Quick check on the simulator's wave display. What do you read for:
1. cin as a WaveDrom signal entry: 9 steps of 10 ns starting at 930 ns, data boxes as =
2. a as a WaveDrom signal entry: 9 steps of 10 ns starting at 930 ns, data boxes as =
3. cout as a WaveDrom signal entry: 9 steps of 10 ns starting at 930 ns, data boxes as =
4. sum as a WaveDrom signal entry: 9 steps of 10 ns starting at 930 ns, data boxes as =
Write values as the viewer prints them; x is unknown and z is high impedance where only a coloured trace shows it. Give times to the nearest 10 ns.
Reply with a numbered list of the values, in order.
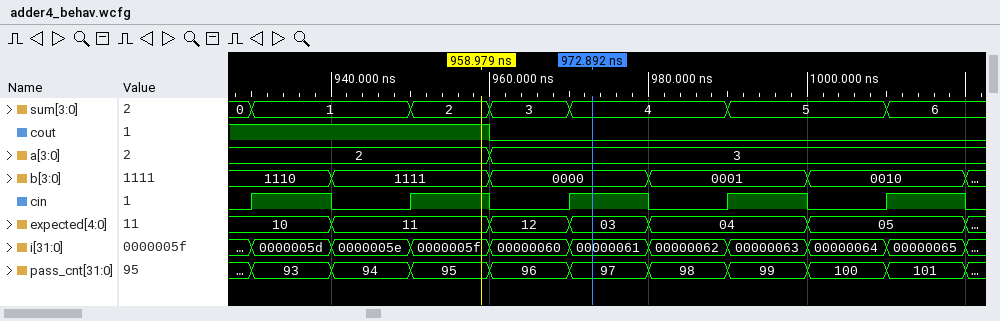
1. {name: 'cin', wave: '101010101'}
2. {name: 'a', wave: '=..=.....', data: '2 3'}
3. {name: 'cout', wave: '1..0.....'}
4. {name: 'sum', wave: '=.===.=.=', data: '1 2 3 4 5 6'}
